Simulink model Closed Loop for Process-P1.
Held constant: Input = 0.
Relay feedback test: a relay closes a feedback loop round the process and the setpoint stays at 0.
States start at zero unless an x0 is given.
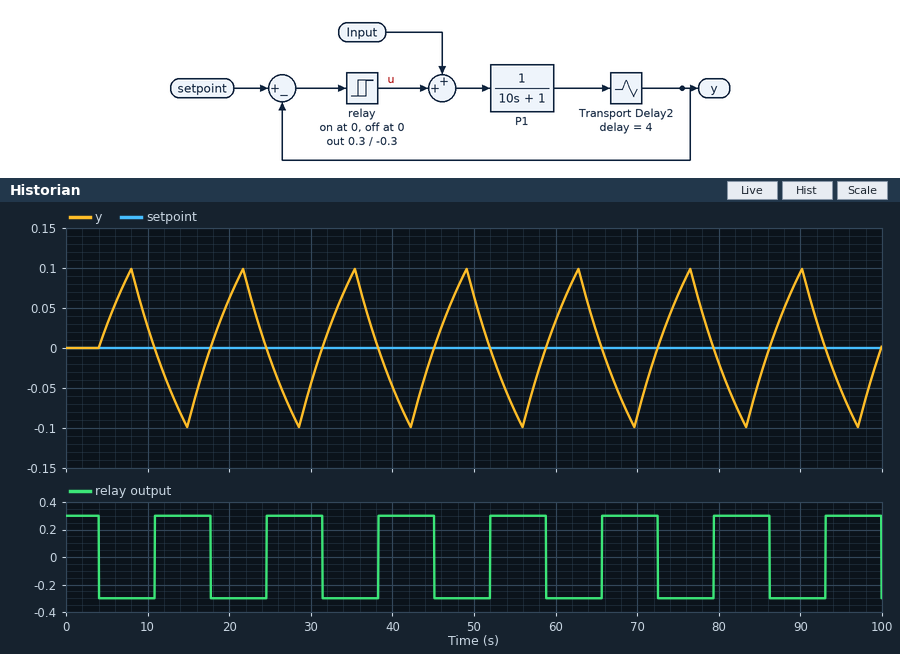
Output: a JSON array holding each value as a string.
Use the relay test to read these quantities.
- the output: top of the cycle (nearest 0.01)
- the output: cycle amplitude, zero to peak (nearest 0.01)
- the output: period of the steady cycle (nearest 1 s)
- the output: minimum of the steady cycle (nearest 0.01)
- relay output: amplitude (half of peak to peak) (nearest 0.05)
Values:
["0.10", "0.10", "14 s", "-0.10", "0.30"]
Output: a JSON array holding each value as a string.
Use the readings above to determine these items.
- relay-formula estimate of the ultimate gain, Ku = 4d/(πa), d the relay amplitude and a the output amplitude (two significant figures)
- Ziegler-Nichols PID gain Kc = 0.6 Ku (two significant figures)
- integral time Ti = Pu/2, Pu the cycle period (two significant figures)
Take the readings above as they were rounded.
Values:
["3.8", "2.3", "7.0 s"]
